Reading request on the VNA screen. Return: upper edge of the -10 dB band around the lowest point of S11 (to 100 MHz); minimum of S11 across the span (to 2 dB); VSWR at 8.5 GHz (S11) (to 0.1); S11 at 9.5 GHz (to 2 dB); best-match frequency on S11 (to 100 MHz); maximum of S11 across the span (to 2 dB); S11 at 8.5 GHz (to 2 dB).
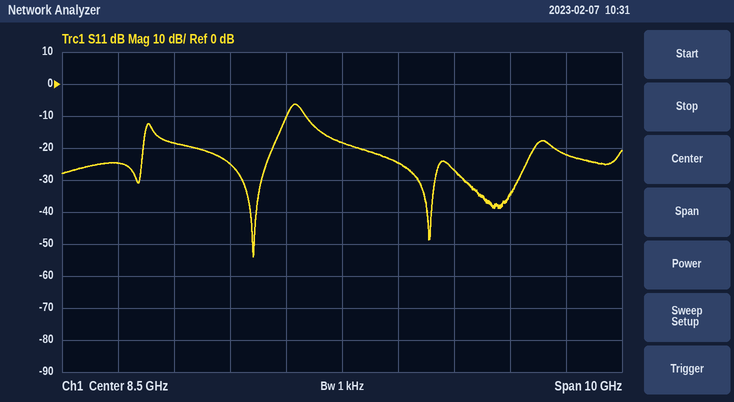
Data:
7.5 GHz
-54 dB
1.3
-24 dB
6.9 GHz
-6 dB
-18 dB
